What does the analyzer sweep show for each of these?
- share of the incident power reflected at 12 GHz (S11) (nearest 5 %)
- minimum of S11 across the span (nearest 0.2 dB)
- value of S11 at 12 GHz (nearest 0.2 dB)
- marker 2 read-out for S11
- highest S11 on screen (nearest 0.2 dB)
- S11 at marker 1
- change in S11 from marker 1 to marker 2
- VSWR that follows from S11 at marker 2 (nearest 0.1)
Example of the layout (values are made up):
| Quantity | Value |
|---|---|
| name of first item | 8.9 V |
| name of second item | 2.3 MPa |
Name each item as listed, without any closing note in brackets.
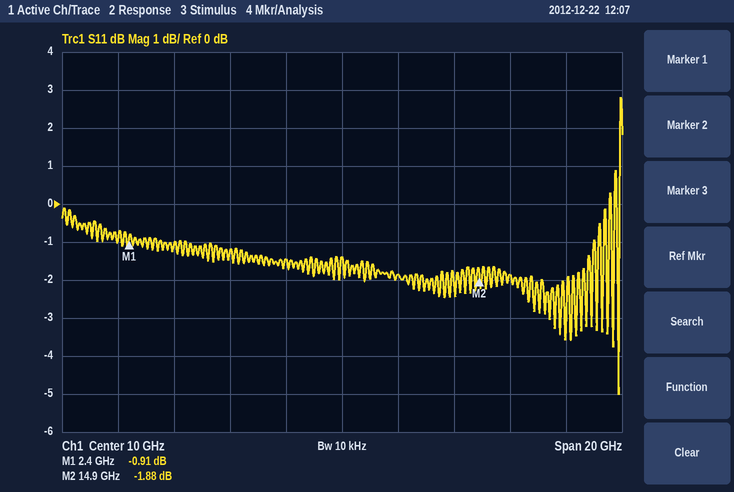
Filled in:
| Quantity | Value |
|---|---|
| share of the incident power reflected at 12 GHz (S11) | 65 % |
| minimum of S11 across the span | -5.0 dB |
| value of S11 at 12 GHz | -1.8 dB |
| marker 2 read-out for S11 | -1.88 dB |
| highest S11 on screen | 2.8 dB |
| S11 at marker 1 | -0.91 dB |
| change in S11 from marker 1 to marker 2 | -0.97 dB |
| VSWR that follows from S11 at marker 2 | 9.3 |
